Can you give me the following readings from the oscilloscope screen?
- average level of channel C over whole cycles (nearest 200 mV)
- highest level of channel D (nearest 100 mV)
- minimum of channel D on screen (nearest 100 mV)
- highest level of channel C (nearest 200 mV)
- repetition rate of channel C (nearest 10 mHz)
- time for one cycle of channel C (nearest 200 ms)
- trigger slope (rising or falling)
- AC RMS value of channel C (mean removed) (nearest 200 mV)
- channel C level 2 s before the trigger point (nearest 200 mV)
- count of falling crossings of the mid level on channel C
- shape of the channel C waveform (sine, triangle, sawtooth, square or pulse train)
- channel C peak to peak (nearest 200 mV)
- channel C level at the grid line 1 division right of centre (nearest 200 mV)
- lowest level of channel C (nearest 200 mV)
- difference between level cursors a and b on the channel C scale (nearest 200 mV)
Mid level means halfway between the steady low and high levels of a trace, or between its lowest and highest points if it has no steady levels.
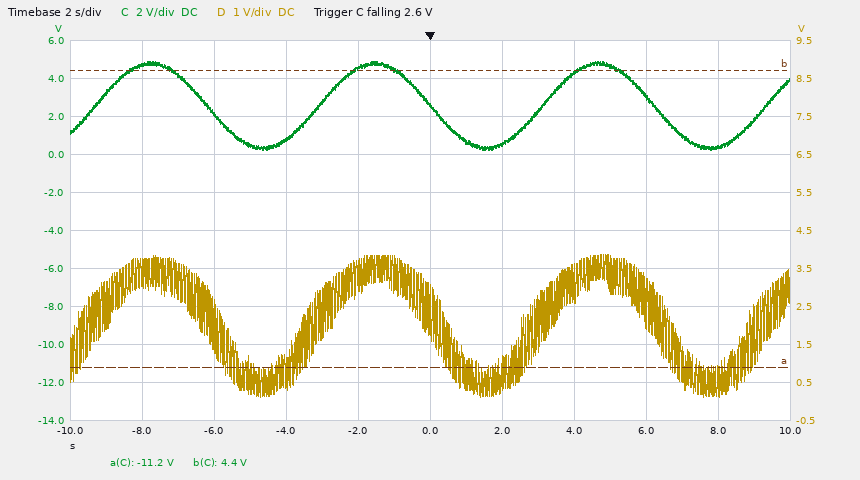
2.6 V
3.9 V
100 mV
4.8 V
160 mHz
6.2 s
falling
1.6 V
4.6 V
3
sine
4.6 V
600 mV
200 mV
15.6 V
